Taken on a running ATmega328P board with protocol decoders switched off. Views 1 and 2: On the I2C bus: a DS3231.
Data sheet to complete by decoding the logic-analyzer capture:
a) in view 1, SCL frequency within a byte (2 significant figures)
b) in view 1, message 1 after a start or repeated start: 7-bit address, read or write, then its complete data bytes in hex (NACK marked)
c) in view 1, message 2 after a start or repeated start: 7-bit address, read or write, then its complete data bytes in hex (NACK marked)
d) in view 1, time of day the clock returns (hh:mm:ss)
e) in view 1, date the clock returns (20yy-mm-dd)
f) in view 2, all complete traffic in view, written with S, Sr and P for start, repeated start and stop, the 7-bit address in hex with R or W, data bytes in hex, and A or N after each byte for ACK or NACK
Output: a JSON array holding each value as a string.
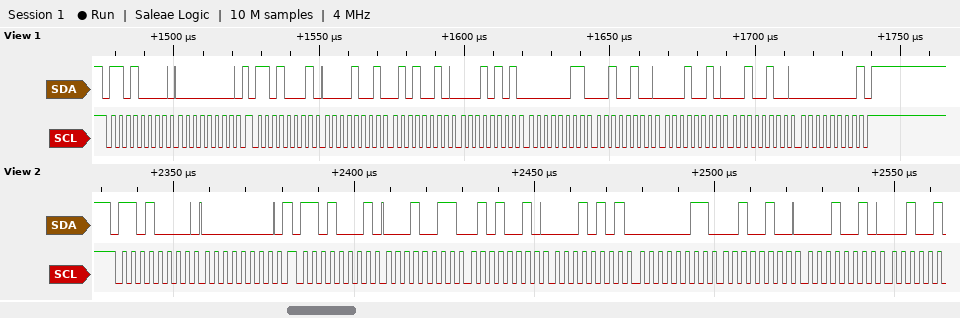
["400 kHz", "0x68 write: 00", "0x68 read: 09 52 15 03 24 12 24 00 NACK", "15:52:09", "2024-12-24", "S 68W A 00 A Sr 68R A 13 A 52 A 15 A 03 A 24 A 12 A"]
